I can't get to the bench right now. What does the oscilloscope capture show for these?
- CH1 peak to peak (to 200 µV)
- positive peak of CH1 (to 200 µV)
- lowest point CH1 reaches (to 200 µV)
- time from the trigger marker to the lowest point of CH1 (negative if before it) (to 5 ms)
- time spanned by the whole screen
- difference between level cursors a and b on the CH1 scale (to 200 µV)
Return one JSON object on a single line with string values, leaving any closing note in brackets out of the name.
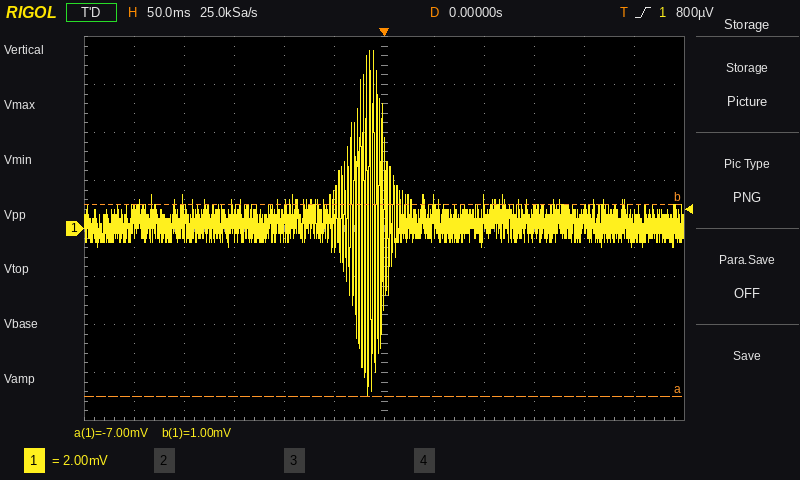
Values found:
{"CH1 peak to peak": "14.4 mV", "positive peak of CH1": "7.4 mV", "lowest point CH1 reaches": "-7.0 mV", "time from the trigger marker to the lowest point of CH1 (negative if before it)": "-15 ms", "time spanned by the whole screen": "600 ms", "difference between level cursors a and b on the CH1 scale": "8.0 mV"}
